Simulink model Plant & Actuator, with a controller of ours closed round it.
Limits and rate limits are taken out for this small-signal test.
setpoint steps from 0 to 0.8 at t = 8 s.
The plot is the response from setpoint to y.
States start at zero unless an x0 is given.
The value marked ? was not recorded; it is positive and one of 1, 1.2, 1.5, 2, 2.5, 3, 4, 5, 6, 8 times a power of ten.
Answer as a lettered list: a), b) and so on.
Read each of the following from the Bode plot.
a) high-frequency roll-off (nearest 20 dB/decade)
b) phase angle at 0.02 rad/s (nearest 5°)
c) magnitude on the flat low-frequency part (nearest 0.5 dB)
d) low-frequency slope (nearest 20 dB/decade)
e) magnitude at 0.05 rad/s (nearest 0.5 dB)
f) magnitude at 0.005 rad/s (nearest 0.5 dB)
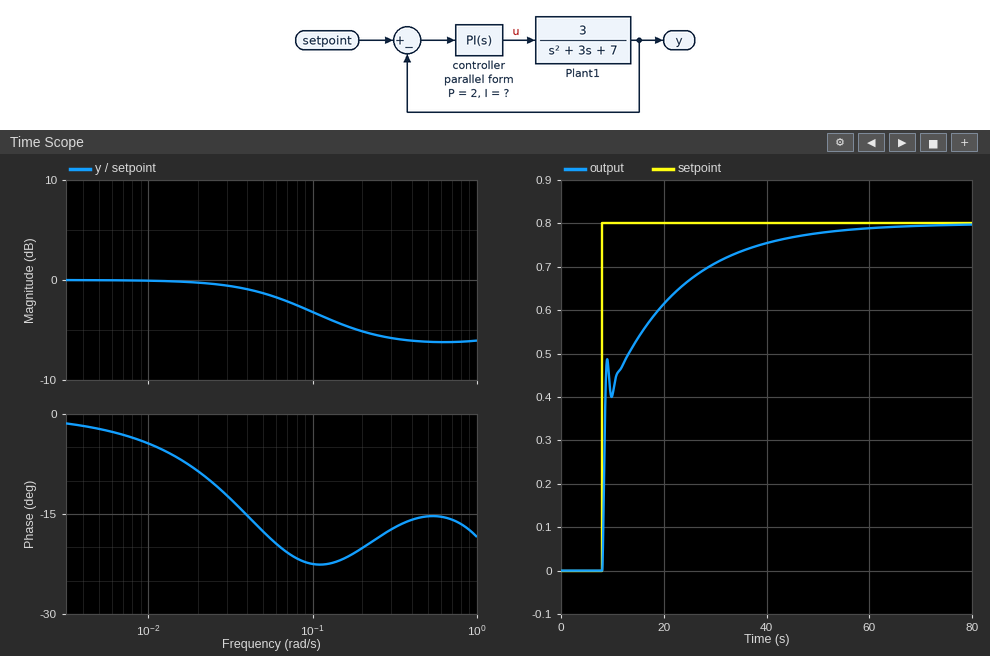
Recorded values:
a) 0 dB/decade
b) -10°
c) 0.0 dB
d) 0 dB/decade
e) -1.5 dB
f) 0.0 dB
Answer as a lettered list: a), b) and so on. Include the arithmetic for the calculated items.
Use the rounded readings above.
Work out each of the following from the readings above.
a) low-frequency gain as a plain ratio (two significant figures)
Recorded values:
a) 10^(0 / 20) = 1.0
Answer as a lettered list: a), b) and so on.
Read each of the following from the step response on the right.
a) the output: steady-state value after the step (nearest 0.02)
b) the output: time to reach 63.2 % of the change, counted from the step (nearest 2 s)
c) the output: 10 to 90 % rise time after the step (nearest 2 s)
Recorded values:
a) 0.80
b) 6 s
c) 24 s
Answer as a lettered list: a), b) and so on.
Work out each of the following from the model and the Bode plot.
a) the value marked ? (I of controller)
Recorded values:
a) 0.3
